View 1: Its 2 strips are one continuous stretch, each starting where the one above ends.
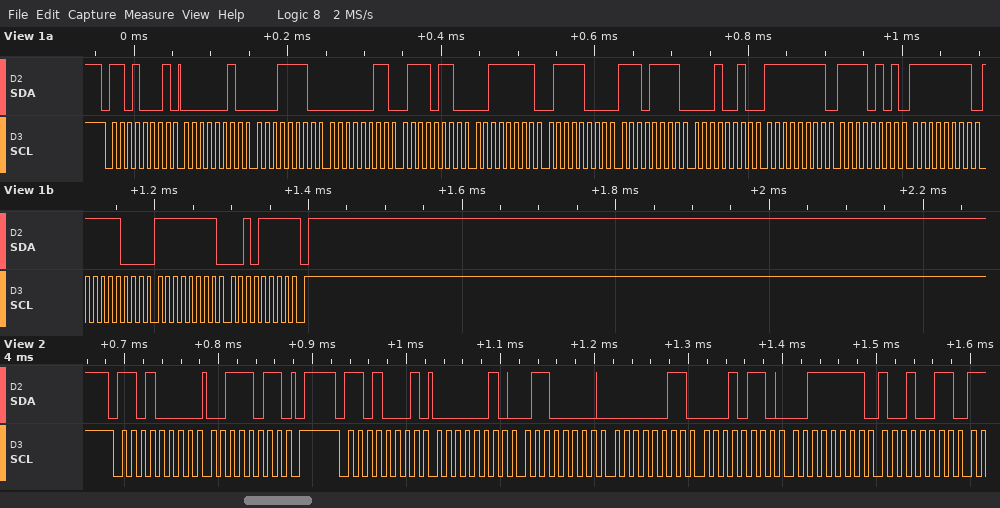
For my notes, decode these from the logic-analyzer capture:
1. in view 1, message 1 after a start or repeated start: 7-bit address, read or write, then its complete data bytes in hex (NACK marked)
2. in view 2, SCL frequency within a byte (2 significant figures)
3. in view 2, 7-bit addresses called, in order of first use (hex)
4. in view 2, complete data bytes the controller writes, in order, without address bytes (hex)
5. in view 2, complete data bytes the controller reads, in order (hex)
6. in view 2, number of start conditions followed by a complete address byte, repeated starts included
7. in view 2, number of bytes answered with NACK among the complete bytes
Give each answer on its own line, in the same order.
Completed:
0x68 read: 02 1E 03 76 3F 78 EF 12 FF F5 FF F8 FF 2F NACK
100 kHz
0x68
3B
02 60 03 16 3F 93
2
0
